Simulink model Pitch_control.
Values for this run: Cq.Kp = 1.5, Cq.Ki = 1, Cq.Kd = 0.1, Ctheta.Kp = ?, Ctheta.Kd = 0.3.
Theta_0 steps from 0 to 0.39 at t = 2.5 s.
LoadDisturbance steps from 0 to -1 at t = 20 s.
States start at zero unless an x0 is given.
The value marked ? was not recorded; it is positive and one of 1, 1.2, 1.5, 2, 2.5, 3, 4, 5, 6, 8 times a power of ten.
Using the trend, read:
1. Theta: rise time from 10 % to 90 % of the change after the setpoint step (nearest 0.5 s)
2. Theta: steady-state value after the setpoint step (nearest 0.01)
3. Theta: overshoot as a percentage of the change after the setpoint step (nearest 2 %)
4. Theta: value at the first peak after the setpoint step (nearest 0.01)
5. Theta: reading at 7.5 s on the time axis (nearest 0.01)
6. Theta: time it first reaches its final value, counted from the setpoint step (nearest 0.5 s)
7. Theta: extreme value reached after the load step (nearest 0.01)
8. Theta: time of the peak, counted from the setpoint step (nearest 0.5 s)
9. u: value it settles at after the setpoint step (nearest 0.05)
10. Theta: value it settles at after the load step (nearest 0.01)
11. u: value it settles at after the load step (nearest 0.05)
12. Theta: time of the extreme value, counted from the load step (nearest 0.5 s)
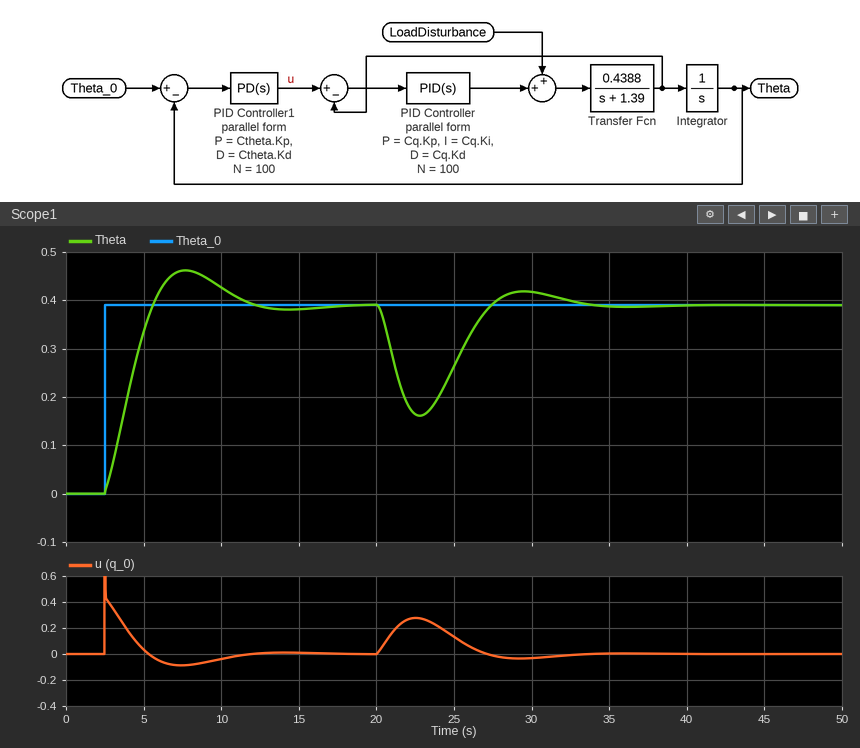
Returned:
2.5 s
0.39
18 %
0.46
0.46
3.0 s
0.16
5.0 s
0.00
0.39
0.00
3.0 s
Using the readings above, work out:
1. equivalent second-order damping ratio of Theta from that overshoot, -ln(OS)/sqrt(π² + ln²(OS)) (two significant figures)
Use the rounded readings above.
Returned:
0.48
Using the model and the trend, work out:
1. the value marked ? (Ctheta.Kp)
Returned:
1.2
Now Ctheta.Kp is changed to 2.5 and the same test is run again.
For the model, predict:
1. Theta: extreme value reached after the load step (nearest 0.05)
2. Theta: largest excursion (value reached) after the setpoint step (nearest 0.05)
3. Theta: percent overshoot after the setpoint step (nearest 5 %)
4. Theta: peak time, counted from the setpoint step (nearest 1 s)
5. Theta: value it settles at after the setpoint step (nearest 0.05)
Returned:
0.25
0.50
25 %
3 s
0.40
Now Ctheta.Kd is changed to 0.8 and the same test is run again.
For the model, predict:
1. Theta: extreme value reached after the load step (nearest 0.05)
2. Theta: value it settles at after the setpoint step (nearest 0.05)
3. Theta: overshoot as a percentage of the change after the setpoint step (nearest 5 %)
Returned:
0.20
0.40
10 %
